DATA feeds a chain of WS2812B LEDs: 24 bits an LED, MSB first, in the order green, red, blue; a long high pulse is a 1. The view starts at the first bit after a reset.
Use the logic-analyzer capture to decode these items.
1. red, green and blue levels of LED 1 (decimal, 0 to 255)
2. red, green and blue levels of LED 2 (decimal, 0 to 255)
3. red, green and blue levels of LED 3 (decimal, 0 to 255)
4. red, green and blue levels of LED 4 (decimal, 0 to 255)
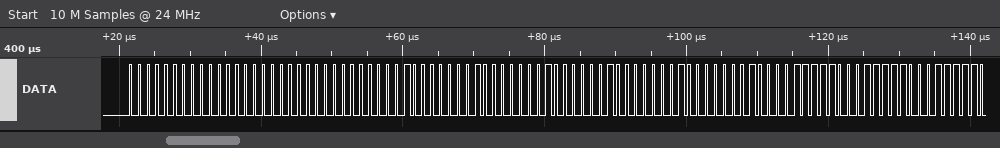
0, 0, 0
1, 1, 1
2, 2, 2
31, 31, 31
